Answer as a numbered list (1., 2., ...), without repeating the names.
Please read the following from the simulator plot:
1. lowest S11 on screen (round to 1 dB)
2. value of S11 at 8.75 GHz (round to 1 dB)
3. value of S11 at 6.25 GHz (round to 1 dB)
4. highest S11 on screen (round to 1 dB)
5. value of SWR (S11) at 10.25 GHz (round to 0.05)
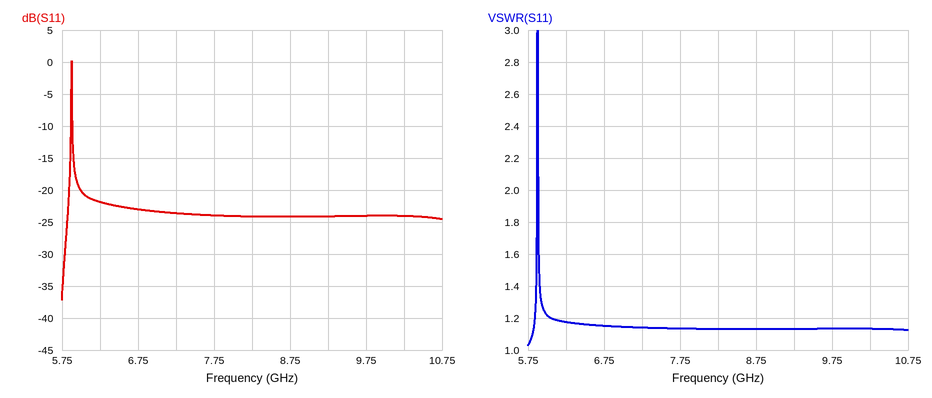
1. -37 dB
2. -24 dB
3. -22 dB
4. 0 dB
5. 1.15
